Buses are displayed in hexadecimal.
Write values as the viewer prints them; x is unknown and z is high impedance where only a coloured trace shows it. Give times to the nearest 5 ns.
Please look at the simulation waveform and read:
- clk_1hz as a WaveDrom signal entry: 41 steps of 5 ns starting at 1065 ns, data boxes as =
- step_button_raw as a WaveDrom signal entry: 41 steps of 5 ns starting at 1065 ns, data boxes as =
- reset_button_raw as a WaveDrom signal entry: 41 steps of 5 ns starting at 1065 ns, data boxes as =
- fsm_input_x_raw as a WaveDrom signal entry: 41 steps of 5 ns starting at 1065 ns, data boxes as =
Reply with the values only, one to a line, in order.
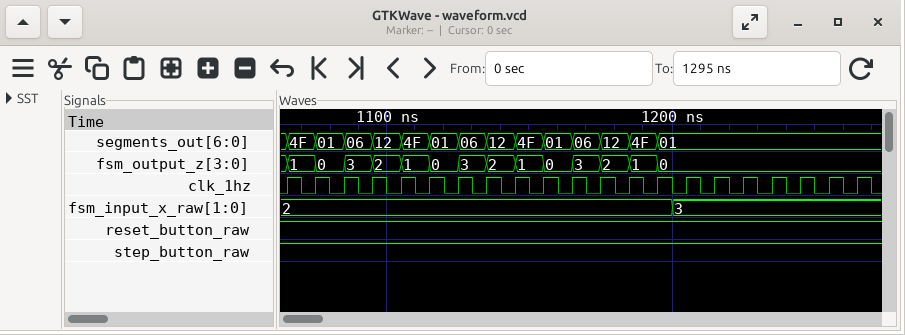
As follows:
{name: 'clk_1hz', wave: '10101010101010101010101010101010101010101'}
{name: 'step_button_raw', wave: '1........................................'}
{name: 'reset_button_raw', wave: '1........................................'}
{name: 'fsm_input_x_raw', wave: '=..........................=.............', data: '2 3'}
